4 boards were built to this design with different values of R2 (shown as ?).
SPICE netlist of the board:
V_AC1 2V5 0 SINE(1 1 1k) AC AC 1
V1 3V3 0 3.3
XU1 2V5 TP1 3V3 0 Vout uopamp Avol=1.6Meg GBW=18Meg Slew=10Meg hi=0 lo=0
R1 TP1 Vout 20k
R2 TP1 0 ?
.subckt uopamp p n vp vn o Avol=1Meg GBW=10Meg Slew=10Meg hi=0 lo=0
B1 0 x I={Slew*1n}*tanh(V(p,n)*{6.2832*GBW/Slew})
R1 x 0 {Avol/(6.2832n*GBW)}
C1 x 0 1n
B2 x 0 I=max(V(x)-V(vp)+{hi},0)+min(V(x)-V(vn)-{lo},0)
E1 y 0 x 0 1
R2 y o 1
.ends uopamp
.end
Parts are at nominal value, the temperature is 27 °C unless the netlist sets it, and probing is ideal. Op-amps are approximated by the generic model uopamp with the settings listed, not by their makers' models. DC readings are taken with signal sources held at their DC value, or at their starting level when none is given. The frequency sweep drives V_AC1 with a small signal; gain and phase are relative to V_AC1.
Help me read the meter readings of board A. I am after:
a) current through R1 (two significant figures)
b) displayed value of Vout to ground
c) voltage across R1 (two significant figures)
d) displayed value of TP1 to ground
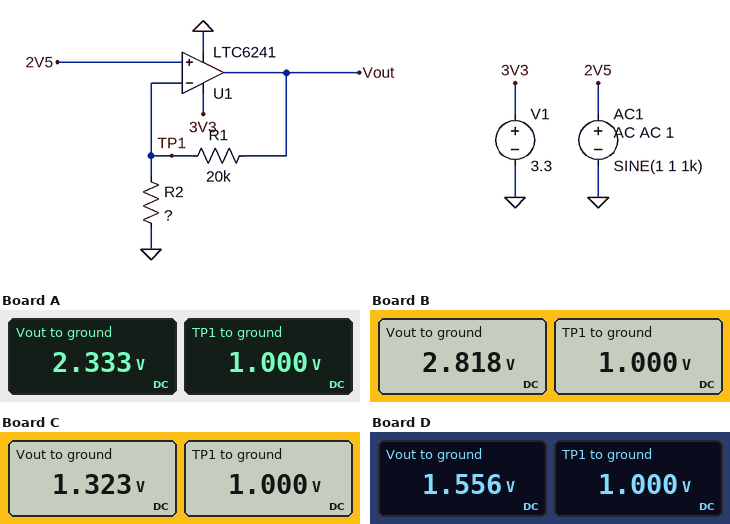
67 µA
2.333 V
1.3 V
1.000 V
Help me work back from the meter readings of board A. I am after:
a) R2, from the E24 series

15 kΩ
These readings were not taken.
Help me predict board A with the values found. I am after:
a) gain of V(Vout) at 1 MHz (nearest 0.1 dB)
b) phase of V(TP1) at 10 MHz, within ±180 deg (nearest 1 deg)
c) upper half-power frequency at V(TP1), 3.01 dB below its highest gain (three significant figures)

7.3 dB
-52 deg
7.71 MHz
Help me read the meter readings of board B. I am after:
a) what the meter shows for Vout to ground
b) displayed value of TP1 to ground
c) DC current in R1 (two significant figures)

2.818 V
1.000 V
91 µA
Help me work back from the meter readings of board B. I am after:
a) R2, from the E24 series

11 kΩ
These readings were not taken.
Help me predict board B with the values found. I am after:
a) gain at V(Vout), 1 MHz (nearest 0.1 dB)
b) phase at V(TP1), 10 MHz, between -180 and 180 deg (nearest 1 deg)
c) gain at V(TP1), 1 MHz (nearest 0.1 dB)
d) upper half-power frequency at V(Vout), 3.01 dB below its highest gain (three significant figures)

8.9 dB
-57 deg
-0.1 dB
6.39 MHz
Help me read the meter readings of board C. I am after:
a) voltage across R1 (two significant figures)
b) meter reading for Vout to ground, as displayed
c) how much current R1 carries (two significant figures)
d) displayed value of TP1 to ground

320 mV
1.323 V
16 µA
1.000 V
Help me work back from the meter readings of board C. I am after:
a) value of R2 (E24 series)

62 kΩ
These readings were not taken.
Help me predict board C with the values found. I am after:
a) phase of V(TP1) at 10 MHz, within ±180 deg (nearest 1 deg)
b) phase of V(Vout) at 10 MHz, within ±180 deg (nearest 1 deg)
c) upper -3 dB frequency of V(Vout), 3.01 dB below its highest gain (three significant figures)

-36 deg
-36 deg
13.6 MHz
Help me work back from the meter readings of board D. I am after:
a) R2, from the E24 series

36 kΩ
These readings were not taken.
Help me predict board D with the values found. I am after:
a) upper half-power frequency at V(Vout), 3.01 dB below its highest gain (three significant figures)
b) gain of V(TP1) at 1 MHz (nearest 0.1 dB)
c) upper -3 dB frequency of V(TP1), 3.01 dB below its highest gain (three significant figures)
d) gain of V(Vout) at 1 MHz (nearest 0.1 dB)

11.6 MHz
0 dB
11.6 MHz
3.8 dB
